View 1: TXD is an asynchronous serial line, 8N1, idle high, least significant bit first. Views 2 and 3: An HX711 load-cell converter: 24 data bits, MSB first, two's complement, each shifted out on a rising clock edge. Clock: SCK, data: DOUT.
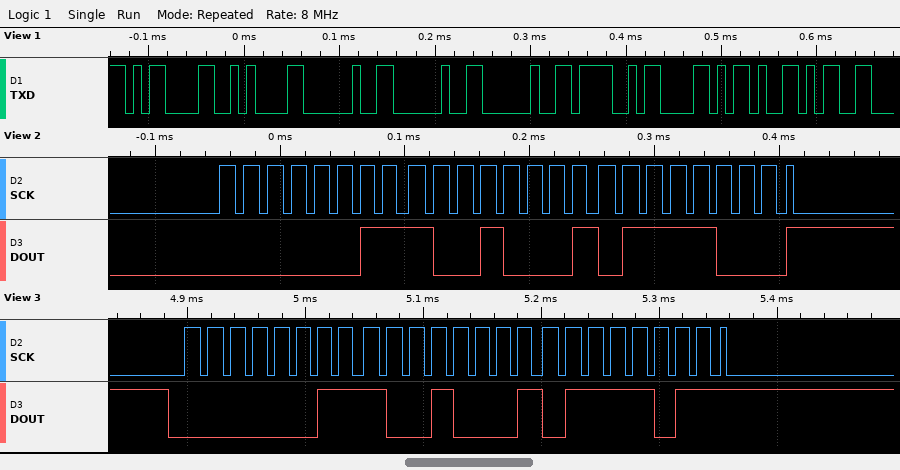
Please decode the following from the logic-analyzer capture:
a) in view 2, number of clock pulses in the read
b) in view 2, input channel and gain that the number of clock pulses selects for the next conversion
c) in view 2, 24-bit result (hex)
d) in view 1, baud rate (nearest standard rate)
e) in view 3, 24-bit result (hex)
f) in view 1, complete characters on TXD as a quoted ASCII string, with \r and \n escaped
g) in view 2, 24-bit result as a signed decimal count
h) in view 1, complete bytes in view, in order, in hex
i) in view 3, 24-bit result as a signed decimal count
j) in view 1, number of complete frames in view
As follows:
25
channel A, gain 128
0x039178
115200 baud
0x03917B
"\r\n   OXY"
233848
0D 0A 20 20 20 4F 58 59
233851
8
